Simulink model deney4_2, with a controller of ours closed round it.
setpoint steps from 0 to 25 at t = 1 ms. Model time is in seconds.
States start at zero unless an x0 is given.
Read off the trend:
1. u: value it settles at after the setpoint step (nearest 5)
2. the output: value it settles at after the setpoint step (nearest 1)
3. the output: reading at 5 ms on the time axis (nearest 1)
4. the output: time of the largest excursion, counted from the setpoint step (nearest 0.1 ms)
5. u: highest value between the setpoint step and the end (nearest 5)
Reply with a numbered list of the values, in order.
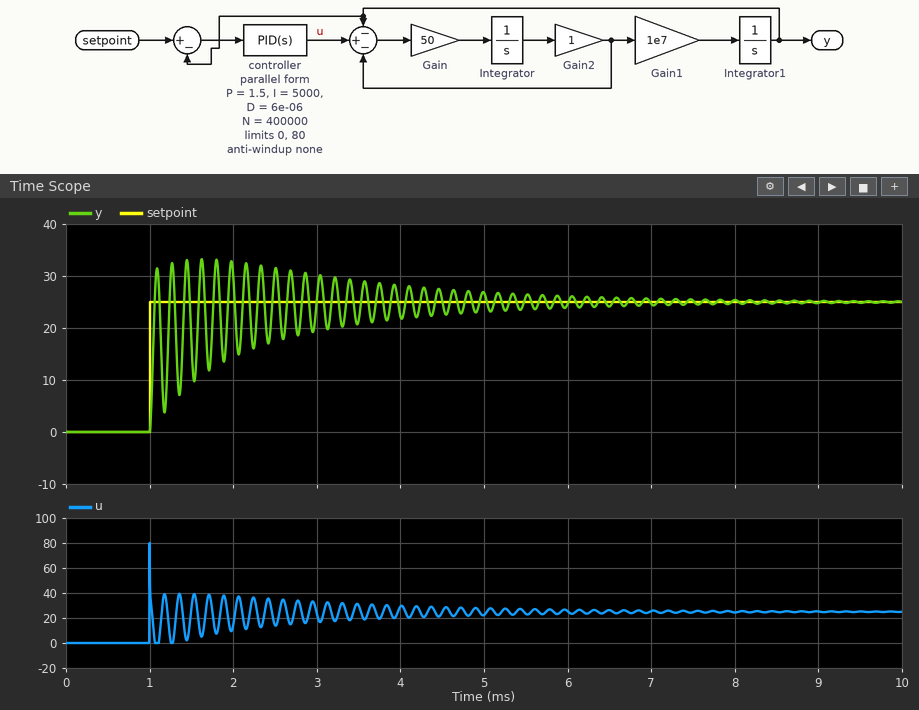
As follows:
1. 25
2. 25
3. 27
4. 0.6 ms
5. 80
